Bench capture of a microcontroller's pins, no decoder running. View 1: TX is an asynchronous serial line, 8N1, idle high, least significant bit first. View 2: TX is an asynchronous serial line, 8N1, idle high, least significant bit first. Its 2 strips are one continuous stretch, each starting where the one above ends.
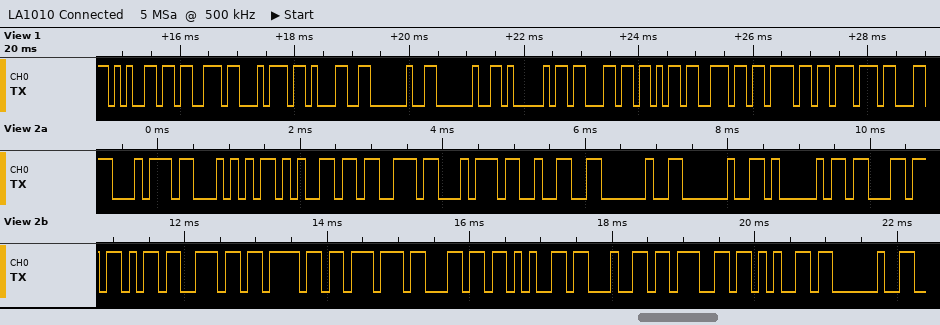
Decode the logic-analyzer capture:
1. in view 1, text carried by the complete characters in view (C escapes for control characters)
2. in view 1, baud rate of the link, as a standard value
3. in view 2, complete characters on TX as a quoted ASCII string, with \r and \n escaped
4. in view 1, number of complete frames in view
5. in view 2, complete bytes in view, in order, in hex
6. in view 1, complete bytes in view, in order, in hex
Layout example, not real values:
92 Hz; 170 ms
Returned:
"est1  Acknow"; 9600 baud; "tTest2  Acknowledge "; 12; 74 54 65 73 74 32 20 20 41 63 6B 6E 6F 77 6C 65 64 67 65 20; 65 73 74 31 20 20 41 63 6B 6E 6F 77
